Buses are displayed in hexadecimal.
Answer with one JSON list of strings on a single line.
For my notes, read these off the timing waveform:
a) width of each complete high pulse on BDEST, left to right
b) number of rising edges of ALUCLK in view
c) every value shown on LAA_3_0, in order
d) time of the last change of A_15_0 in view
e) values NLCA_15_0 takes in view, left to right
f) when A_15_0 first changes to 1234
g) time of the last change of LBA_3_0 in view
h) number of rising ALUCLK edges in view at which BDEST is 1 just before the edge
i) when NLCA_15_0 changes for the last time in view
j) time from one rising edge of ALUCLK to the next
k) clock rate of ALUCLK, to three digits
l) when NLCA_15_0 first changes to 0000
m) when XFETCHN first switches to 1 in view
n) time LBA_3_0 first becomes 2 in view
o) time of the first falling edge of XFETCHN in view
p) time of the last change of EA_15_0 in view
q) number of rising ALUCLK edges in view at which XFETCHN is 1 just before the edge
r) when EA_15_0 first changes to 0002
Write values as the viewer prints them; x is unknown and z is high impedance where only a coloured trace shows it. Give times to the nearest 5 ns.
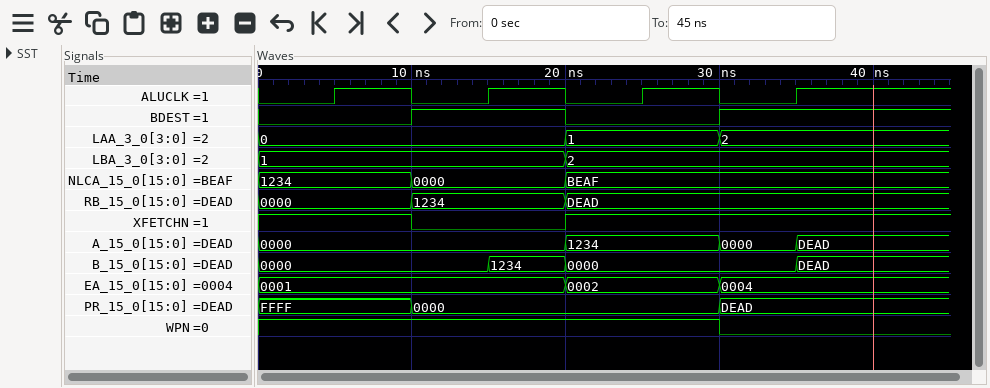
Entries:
["10 ns", "4", "0, 1, 2", "35 ns", "1234, 0000, BEAF", "20 ns", "20 ns", "2", "20 ns", "10 ns", "100 MHz", "10 ns", "20 ns", "20 ns", "10 ns", "30 ns", "3", "20 ns"]
